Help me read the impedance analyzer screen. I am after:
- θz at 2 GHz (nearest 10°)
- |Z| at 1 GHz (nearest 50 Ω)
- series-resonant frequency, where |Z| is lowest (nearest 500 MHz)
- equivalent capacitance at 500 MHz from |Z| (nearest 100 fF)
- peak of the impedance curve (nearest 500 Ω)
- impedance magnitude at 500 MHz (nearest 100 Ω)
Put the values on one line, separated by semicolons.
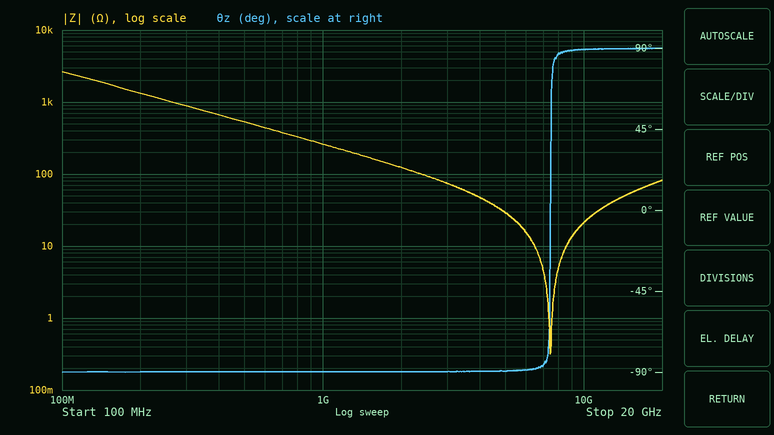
-90°; 250 Ω; 7.5 GHz; 600 fF; 2.5 kΩ; 500 Ω
